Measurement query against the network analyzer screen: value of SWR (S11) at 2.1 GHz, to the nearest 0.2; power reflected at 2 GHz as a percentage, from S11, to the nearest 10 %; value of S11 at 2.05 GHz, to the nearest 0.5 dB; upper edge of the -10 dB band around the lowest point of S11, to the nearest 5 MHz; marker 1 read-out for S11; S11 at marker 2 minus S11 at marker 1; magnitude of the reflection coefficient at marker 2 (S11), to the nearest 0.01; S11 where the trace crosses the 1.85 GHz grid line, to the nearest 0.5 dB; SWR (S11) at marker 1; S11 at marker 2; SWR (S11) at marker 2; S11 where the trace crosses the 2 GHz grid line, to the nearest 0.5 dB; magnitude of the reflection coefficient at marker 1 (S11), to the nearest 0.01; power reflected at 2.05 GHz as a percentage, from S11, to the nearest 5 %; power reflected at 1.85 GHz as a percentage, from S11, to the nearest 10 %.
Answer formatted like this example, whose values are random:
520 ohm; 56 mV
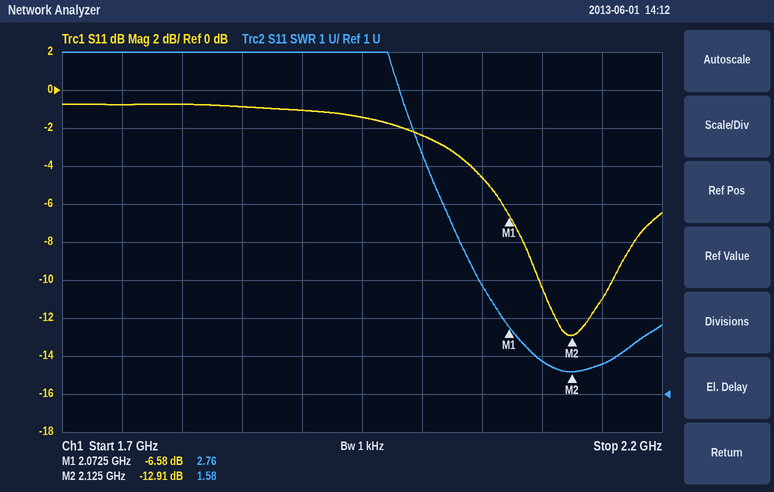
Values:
1.8; 60 %; -4.5 dB; 2.160 GHz; -6.58 dB; -6.33 dB; 0.23; -1.0 dB; 2.76; -12.91 dB; 1.58; -2.5 dB; 0.47; 35 %; 80 %
